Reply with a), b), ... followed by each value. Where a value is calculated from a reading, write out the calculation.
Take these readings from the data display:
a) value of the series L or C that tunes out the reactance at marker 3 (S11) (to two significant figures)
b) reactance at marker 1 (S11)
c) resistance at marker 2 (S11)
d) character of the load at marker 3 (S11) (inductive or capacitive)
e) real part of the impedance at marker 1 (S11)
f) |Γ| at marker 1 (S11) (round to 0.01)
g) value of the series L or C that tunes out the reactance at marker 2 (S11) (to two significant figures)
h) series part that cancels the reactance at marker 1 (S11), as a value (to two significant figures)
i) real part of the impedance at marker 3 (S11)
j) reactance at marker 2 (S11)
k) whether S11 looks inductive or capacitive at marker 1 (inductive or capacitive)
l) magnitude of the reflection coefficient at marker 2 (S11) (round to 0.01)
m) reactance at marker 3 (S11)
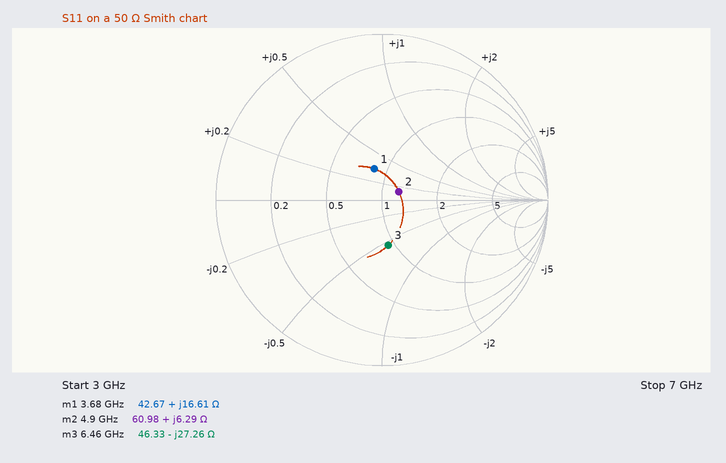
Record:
a) L = 27.26 Ω/(2π × 6.46 GHz) ≈ 672 pH, so 670 pH to two significant figures
b) +16.61 Ω
c) 60.98 Ω
d) capacitive
e) 42.67 Ω
f) 0.19
g) C = 1/(2π × 4.9 GHz × 6.29 Ω) ≈ 5.2 pF
h) C = 1/(2π × 3.68 GHz × 16.61 Ω) ≈ 2.6 pF
i) 46.33 Ω
j) +6.29 Ω
k) inductive
l) 0.11
m) -27.26 Ω
